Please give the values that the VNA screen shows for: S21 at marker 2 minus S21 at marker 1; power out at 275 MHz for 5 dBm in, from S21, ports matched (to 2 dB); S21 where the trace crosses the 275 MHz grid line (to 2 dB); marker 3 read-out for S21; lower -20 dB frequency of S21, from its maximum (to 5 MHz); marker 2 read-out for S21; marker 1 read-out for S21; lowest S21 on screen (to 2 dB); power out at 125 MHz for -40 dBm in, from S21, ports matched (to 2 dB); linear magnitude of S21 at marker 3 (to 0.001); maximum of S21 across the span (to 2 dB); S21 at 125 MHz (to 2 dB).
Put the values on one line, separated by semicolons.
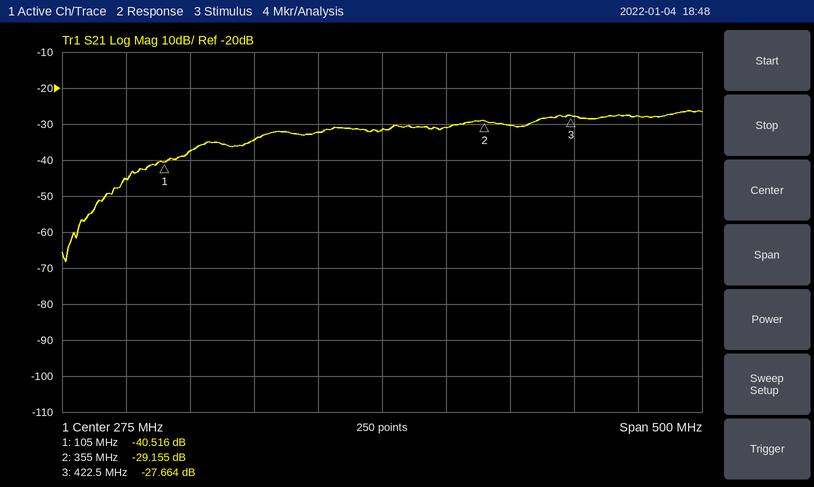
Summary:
11.361 dB; -26 dBm; -32 dB; -27.664 dB; 70 MHz; -29.155 dB; -40.516 dB; -68 dB; -78 dBm; 0.041; -26 dB; -38 dB
